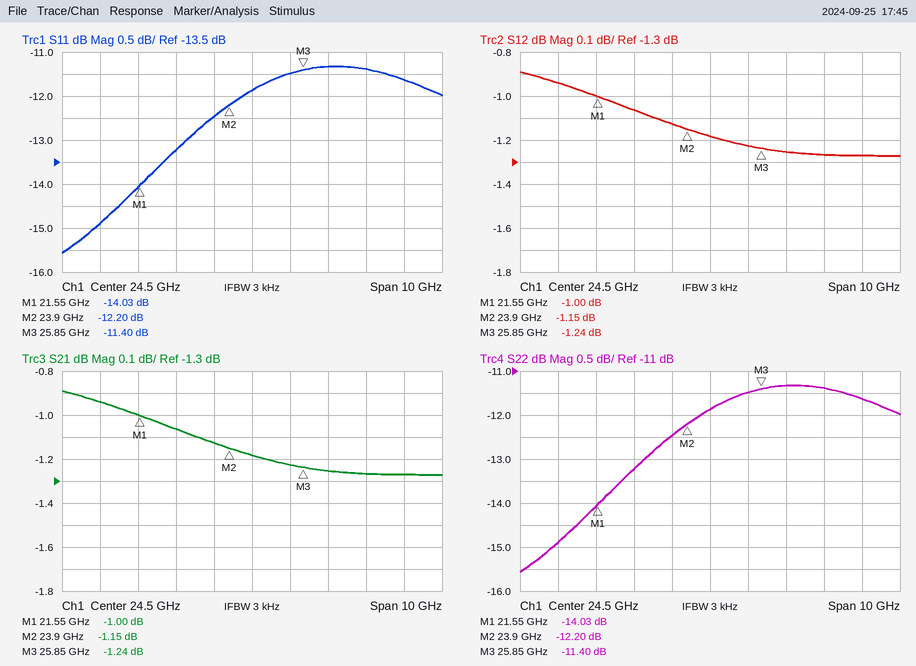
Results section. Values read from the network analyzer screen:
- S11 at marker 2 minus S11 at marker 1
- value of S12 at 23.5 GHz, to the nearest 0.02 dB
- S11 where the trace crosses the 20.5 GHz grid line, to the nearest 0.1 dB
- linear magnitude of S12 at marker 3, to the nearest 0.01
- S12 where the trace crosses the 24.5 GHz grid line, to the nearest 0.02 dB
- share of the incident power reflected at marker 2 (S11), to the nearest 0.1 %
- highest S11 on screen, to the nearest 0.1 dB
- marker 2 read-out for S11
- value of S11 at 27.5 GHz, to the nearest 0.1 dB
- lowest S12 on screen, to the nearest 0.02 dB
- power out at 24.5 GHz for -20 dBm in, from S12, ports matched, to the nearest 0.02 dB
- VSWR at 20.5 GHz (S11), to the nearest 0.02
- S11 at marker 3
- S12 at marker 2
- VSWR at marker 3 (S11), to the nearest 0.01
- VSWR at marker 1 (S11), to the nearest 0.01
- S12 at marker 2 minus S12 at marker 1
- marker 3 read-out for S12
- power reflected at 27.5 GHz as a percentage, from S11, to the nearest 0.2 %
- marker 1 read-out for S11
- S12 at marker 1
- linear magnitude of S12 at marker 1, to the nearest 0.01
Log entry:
1.83 dB
-1.12 dB
-14.9 dB
0.87
-1.18 dB
6.0 %
-11.3 dB
-12.20 dB
-11.4 dB
-1.28 dB
-21.18 dBm
1.44
-11.40 dB
-1.15 dB
1.74
1.50
-0.15 dB
-1.24 dB
7.2 %
-14.03 dB
-1.00 dB
0.89
